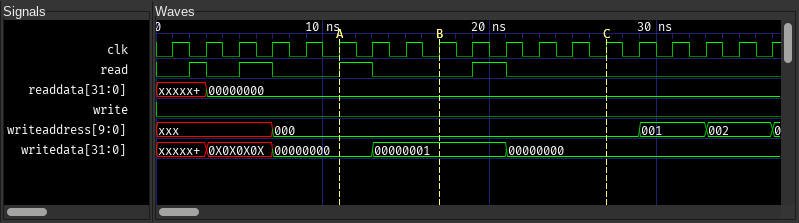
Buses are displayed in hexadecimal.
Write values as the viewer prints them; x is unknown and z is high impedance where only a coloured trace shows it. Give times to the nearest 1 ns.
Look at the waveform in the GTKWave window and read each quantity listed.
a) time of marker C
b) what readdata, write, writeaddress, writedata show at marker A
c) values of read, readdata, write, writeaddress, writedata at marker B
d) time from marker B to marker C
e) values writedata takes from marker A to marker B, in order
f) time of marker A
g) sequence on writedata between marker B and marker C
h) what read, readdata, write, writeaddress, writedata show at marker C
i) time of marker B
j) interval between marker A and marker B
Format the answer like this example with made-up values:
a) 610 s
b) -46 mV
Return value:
a) 27 ns
b) readdata=00000000, write=0, writeaddress=000, writedata=00000000
c) read=0, readdata=00000000, write=0, writeaddress=000, writedata=00000001
d) 10 ns
e) 00000000, 00000001
f) 11 ns
g) 00000001, 00000000
h) read=0, readdata=00000000, write=0, writeaddress=000, writedata=00000000
i) 17 ns
j) 6 ns
